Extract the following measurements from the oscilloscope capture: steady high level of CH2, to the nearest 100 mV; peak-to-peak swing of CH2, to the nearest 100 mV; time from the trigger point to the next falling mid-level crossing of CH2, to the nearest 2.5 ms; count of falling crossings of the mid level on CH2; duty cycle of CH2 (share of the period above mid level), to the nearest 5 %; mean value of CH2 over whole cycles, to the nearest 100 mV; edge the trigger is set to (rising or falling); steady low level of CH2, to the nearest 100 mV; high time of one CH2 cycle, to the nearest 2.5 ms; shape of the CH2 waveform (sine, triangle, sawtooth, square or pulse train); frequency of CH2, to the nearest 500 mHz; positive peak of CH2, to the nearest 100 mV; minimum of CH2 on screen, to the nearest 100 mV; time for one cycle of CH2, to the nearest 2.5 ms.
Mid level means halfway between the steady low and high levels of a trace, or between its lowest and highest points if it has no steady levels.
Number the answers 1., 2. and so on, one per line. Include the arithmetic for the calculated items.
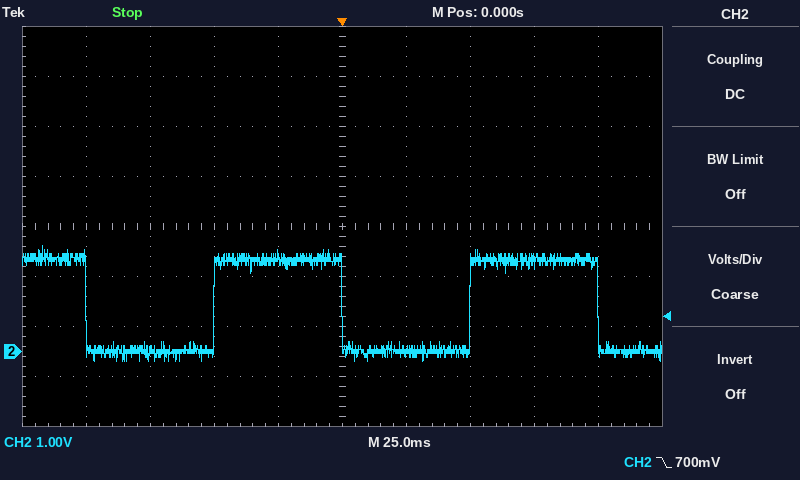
1. 1.8 V
2. 2.1 V − (-200 mV) = 2.3 V
3. 100.0 ms
4. 3
5. 50.0 ms / 100.0 ms ≈ 50 %
6. 0.0 V + 0.5 × (1.8 V − (0.0 V)) ≈ 900 mV
7. falling
8. 0.0 V
9. 50.0 ms
10. square
11. 1 / 100.0 ms ≈ 10.0 Hz
12. 2.1 V
13. -200 mV
14. 100.0 ms
